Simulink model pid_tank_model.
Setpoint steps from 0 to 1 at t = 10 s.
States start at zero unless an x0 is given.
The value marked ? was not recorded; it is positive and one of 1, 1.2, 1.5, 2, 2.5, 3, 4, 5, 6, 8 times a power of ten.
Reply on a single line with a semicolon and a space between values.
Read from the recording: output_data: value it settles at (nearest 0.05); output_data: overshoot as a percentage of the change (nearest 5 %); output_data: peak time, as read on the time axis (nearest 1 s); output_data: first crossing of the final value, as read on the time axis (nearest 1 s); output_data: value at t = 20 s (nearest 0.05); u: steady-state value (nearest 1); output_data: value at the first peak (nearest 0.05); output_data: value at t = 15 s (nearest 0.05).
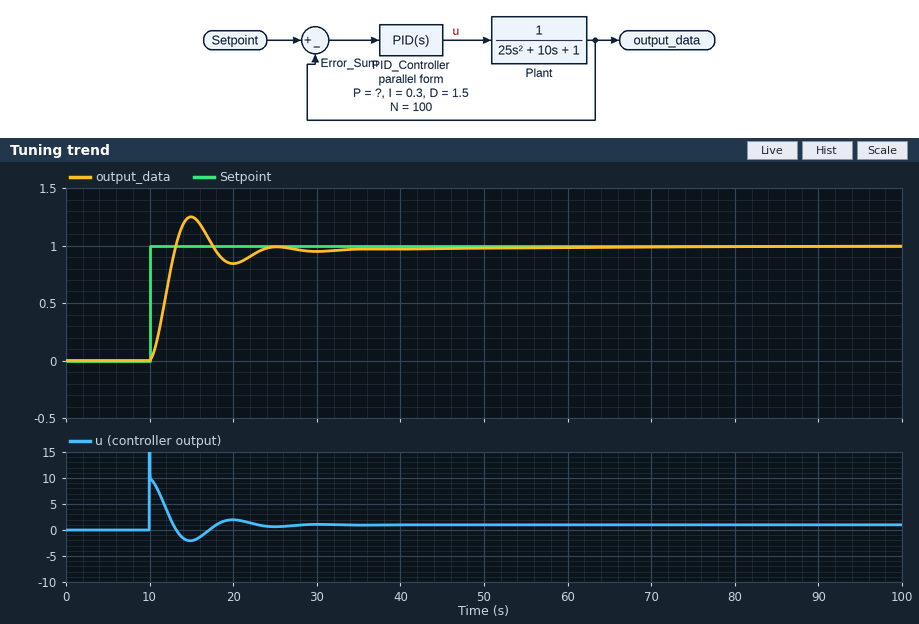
1.00; 25 %; 15 s; 13 s; 0.85; 1; 1.25; 1.25
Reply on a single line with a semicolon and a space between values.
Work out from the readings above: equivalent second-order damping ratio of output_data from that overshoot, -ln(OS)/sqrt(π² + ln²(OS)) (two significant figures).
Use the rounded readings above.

0.40
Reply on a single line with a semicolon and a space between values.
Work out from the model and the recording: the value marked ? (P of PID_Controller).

10
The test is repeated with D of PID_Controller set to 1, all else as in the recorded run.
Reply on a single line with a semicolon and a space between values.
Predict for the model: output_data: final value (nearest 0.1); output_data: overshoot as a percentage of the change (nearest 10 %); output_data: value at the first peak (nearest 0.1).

1.0; 30 %; 1.3
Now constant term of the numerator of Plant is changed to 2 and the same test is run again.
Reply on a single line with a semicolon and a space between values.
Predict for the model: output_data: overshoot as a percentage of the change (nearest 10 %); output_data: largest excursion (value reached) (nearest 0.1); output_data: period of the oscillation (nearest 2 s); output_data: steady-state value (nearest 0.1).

40 %; 1.4; 8 s; 1.0
